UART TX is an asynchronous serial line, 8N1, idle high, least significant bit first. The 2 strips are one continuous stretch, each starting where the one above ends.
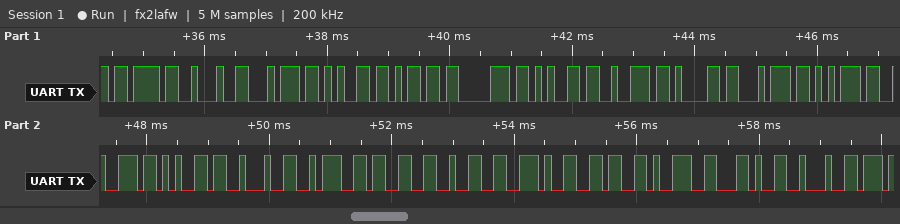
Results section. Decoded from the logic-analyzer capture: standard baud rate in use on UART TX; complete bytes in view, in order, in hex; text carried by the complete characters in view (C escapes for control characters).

9600 baud
7B 22 74 65 6D 70 65 72 61 74 75 72 65 22 3A 33 32 2E 36 39 2C 22
"{\"temperature\":32.69,\""
